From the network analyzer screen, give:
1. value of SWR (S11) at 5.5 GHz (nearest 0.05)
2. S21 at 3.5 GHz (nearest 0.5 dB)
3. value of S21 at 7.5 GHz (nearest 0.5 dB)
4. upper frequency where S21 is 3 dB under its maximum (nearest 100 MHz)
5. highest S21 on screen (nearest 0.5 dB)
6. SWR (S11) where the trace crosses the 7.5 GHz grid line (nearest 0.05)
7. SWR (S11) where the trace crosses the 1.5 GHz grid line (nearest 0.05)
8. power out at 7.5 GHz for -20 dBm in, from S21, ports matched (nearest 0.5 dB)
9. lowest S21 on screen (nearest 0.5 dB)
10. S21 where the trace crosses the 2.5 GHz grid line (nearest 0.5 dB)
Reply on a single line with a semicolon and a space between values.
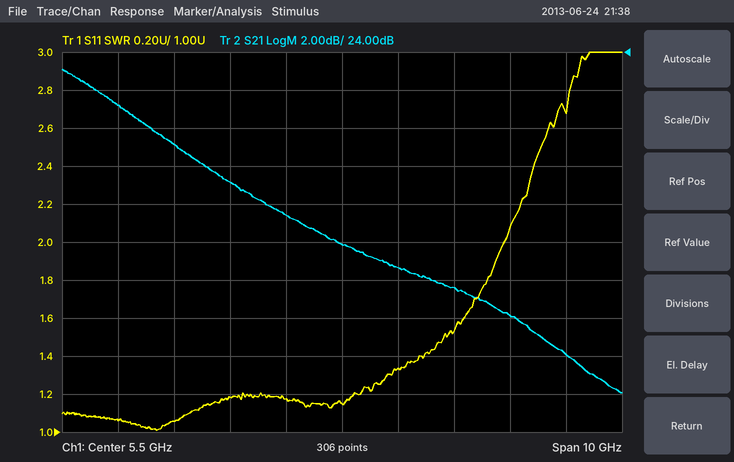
1.15; 17.0 dB; 11.5 dB; 2.0 GHz; 23.0 dB; 1.55; 1.05; -8.5 dBm; 6.0 dB; 19.0 dB
